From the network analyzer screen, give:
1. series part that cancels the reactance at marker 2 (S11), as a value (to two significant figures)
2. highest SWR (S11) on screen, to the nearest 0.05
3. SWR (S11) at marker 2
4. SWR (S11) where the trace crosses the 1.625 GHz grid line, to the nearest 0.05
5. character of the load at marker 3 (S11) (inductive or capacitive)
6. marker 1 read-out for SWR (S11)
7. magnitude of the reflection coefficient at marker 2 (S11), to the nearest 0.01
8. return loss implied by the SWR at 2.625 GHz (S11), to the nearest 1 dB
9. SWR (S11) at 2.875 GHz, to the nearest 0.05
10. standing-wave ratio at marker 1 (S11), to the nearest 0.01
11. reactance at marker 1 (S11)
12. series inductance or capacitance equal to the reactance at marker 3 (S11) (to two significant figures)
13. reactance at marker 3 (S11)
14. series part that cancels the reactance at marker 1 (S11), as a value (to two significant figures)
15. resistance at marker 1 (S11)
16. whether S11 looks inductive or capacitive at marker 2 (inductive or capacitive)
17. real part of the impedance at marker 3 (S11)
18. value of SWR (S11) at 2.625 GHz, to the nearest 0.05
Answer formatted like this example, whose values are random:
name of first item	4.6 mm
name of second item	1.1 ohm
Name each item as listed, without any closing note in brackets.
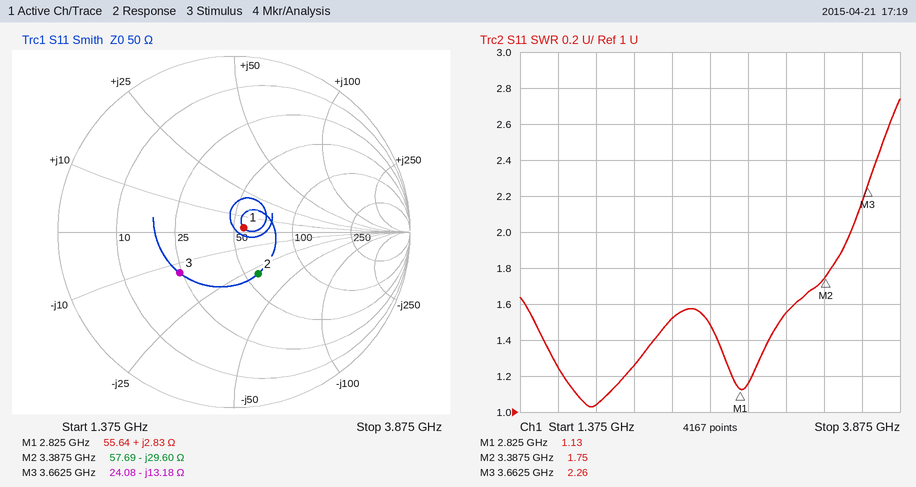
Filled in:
series part that cancels the reactance at marker 2 (S11), as a value	1.4 nH
highest SWR (S11) on screen, to the nearest 0.05	2.75
SWR (S11) at marker 2	1.75
SWR (S11) where the trace crosses the 1.625 GHz grid line, to the nearest 0.05	1.25
character of the load at marker 3 (S11)	capacitive
marker 1 read-out for SWR	1.13
magnitude of the reflection coefficient at marker 2 (S11), to the nearest 0.01	0.27
return loss implied by the SWR at 2.625 GHz (S11), to the nearest 1 dB	14 dB
SWR (S11) at 2.875 GHz, to the nearest 0.05	1.15
standing-wave ratio at marker 1 (S11), to the nearest 0.01	1.13
reactance at marker 1	+2.83 Ω
series inductance or capacitance equal to the reactance at marker 3 (S11)	3.3 pF
reactance at marker 3	-13.18 Ω
series part that cancels the reactance at marker 1 (S11), as a value	20 pF
resistance at marker 1	55.64 Ω
whether S11 looks inductive or capacitive at marker 2	capacitive
real part of the impedance at marker 3	24.08 Ω
value of SWR (S11) at 2.625 GHz, to the nearest 0.05	1.50
